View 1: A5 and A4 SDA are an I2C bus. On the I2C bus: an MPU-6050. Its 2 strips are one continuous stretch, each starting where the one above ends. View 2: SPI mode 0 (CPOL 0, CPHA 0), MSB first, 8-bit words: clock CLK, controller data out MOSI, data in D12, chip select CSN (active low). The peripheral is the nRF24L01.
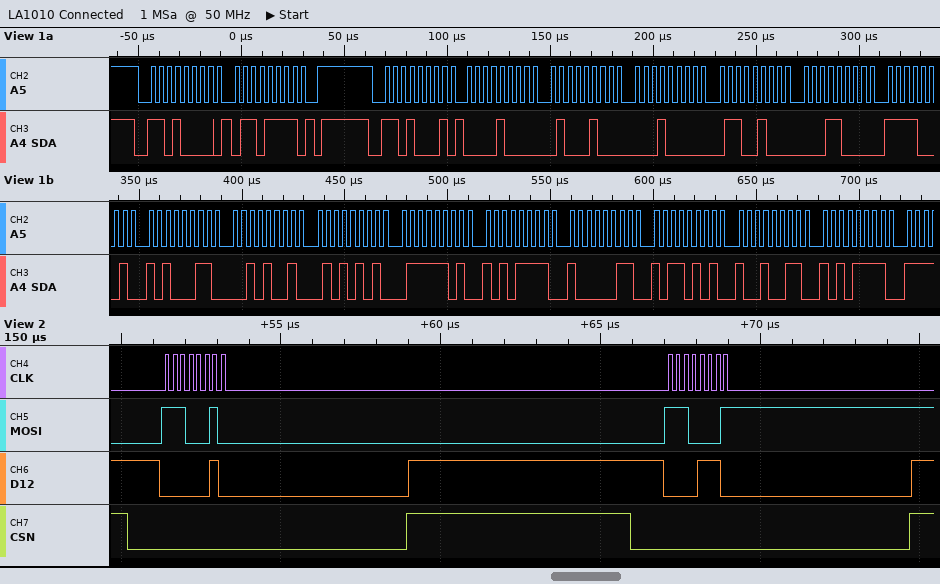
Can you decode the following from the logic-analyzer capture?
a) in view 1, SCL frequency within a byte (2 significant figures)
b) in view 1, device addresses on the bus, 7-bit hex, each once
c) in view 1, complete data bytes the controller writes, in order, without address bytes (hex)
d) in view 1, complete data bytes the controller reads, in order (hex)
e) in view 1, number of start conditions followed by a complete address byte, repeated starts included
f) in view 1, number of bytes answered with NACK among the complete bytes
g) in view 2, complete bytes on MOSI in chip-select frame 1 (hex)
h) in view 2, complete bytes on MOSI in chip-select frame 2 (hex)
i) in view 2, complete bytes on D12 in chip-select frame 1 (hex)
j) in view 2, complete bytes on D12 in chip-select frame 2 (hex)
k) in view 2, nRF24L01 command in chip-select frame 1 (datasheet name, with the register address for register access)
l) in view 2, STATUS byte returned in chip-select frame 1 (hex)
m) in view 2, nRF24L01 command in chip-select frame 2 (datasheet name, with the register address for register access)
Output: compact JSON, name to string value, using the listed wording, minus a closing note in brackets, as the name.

{"in view 1, SCL frequency within a byte": "250 kHz", "in view 1, device addresses on the bus, 7-bit hex, each once": "0x68", "in view 1, complete data bytes the controller writes, in order, without address bytes": "6F", "in view 1, complete data bytes the controller reads, in order": "08 44 10 64 18 F1 A3 29 55 7D AF 83 B5 93 AF", "in view 1, number of start conditions followed by a complete address byte, repeated starts included": "2", "in view 1, number of bytes answered with NACK among the complete bytes": "0", "in view 2, complete bytes on MOSI in chip-select frame 1": "E2", "in view 2, complete bytes on MOSI in chip-select frame 2": "E1", "in view 2, complete bytes on D12 in chip-select frame 1": "02", "in view 2, complete bytes on D12 in chip-select frame 2": "0E", "in view 2, nRF24L01 command in chip-select frame 1": "FLUSH_RX", "in view 2, STATUS byte returned in chip-select frame 1": "0x02", "in view 2, nRF24L01 command in chip-select frame 2": "FLUSH_TX"}
